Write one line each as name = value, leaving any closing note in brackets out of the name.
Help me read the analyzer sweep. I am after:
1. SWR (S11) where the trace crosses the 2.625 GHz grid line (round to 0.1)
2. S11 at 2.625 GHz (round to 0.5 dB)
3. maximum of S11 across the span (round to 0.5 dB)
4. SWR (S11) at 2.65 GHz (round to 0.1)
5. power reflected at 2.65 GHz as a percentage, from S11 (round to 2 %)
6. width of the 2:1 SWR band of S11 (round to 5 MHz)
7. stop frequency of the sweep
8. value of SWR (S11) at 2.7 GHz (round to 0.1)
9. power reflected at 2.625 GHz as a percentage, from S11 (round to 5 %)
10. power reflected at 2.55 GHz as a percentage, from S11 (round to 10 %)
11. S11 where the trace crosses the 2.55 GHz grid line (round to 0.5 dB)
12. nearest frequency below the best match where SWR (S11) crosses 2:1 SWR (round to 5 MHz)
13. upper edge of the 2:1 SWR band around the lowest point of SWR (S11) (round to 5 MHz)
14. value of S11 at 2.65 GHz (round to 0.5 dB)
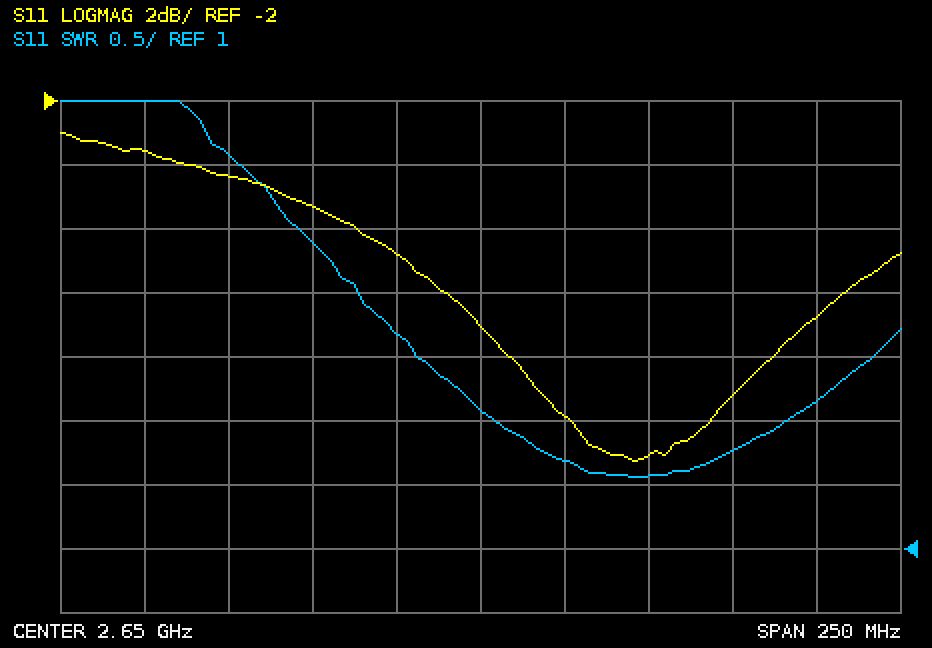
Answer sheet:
SWR (S11) where the trace crosses the 2.625 GHz grid line = 2.7
S11 at 2.625 GHz = -7.0 dB
maximum of S11 across the span = -3.0 dB
SWR (S11) at 2.65 GHz = 2.1
power reflected at 2.65 GHz as a percentage, from S11 = 12 %
width of the 2:1 SWR band of S11 = 85 MHz
stop frequency of the sweep = 2.775 GHz
value of SWR (S11) at 2.7 GHz = 1.6
power reflected at 2.625 GHz as a percentage, from S11 = 20 %
power reflected at 2.55 GHz as a percentage, from S11 = 40 %
S11 where the trace crosses the 2.55 GHz grid line = -3.5 dB
nearest frequency below the best match where SWR (S11) crosses 2:1 SWR = 2.655 GHz
upper edge of the 2:1 SWR band around the lowest point of SWR (S11) = 2.740 GHz
value of S11 at 2.65 GHz = -9.0 dB
